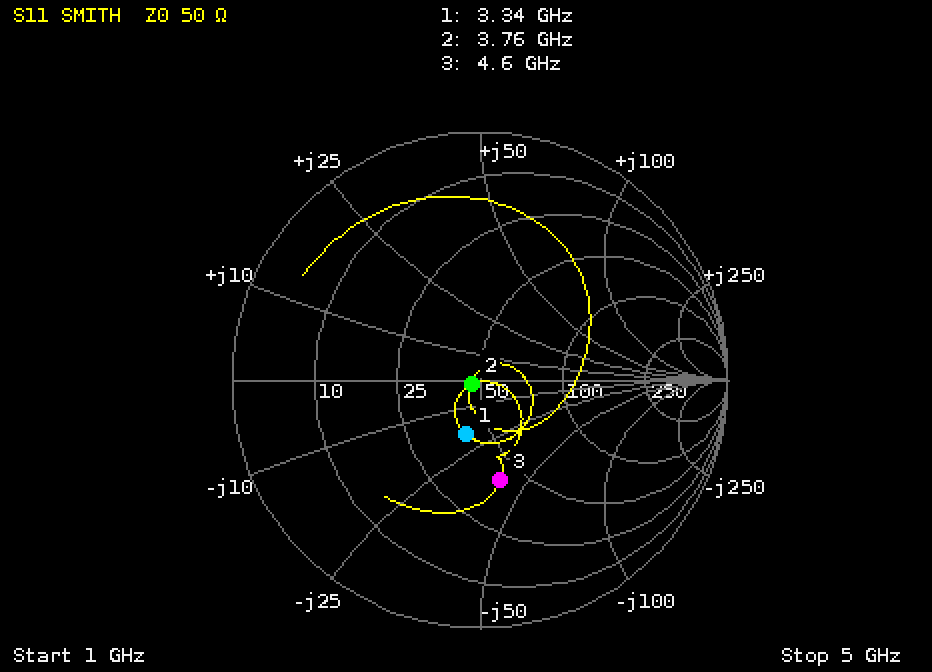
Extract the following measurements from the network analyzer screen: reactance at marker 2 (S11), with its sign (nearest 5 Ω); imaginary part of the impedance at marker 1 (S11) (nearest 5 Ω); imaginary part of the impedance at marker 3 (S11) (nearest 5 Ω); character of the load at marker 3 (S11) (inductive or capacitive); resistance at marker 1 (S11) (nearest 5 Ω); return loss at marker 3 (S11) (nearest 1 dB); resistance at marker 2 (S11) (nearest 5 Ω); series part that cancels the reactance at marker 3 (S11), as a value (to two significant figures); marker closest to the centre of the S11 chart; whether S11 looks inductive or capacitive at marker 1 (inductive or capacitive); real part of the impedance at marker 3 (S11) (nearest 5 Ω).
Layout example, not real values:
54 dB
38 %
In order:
0 Ω
-20 Ω
-40 Ω
capacitive
40 Ω
8 dB
45 Ω
1.4 nH
marker 2
capacitive
40 Ω
